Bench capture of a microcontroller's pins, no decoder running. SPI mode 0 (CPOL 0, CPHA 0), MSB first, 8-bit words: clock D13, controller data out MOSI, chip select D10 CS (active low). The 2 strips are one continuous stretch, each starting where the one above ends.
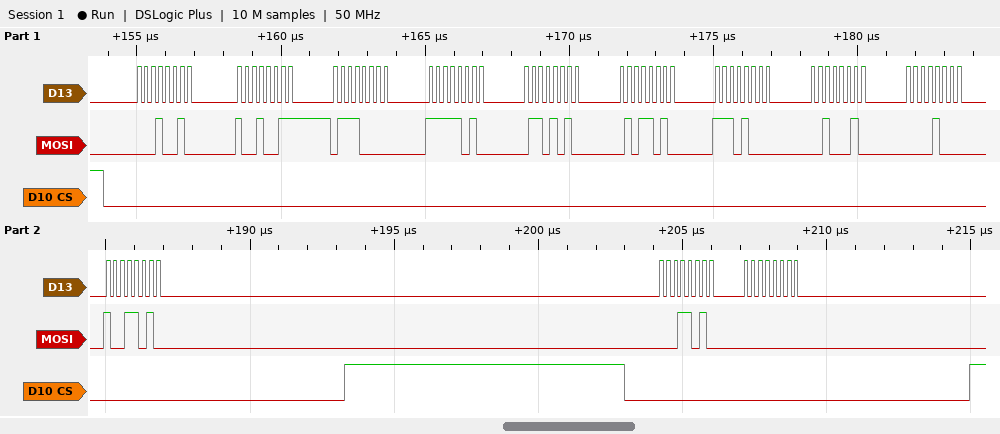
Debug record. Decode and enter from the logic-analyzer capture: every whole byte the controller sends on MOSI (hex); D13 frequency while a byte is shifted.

12 93 70 FA 6A 5A E8 22 08 9A 1A 00
4 MHz
